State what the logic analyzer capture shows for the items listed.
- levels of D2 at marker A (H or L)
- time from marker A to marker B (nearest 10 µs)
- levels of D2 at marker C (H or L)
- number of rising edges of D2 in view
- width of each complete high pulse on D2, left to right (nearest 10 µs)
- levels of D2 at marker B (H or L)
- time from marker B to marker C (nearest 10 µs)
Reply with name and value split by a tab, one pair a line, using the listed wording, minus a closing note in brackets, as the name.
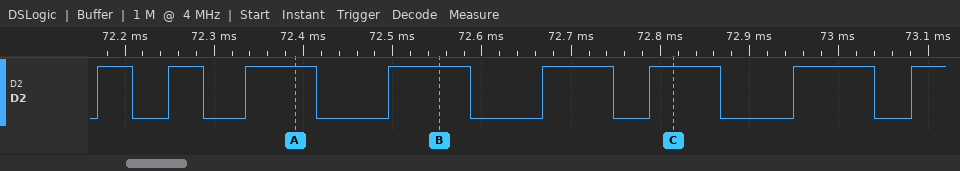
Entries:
levels of D2 at marker A	D2=H
time from marker A to marker B	160 µs
levels of D2 at marker C	D2=H
number of rising edges of D2 in view	8
width of each complete high pulse on D2, left to right	40 µs, 40 µs, 80 µs, 90 µs, 80 µs, 80 µs, 90 µs
levels of D2 at marker B	D2=H
time from marker B to marker C	260 µs
